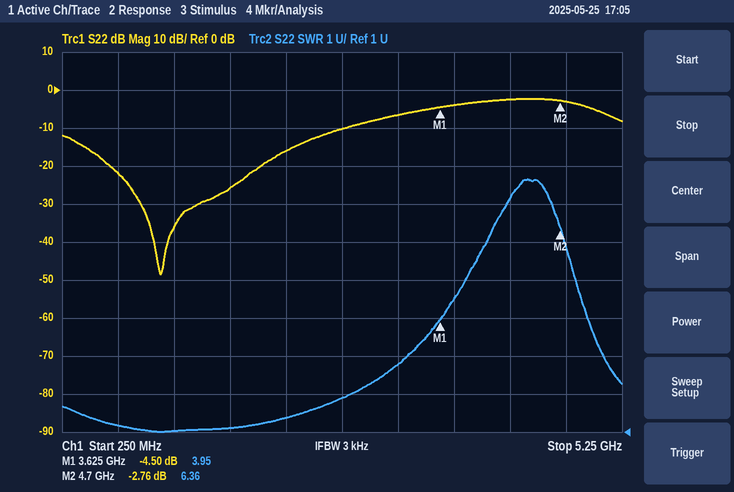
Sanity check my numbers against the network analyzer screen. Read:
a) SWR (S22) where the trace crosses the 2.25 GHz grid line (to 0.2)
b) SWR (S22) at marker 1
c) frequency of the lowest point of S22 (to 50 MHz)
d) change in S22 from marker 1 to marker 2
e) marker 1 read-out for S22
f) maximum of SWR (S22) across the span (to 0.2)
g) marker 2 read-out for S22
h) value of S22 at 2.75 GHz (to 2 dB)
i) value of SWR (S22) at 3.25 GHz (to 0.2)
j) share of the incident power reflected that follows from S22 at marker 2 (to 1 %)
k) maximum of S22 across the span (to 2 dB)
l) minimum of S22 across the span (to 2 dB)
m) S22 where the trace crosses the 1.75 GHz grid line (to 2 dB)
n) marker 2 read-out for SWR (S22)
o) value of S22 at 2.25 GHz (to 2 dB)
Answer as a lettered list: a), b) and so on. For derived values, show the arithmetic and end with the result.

a) 1.4
b) 3.95
c) 1.15 GHz
d) -2.76 − (-4.5) = 1.74 dB
e) -4.50 dB
f) 7.6
g) -2.76 dB
h) -10 dB
i) 2.8
j) 10^(-2.76/10) ≈ 53 %
k) -2 dB
l) -48 dB
m) -26 dB
n) 6.36
o) -16 dB
